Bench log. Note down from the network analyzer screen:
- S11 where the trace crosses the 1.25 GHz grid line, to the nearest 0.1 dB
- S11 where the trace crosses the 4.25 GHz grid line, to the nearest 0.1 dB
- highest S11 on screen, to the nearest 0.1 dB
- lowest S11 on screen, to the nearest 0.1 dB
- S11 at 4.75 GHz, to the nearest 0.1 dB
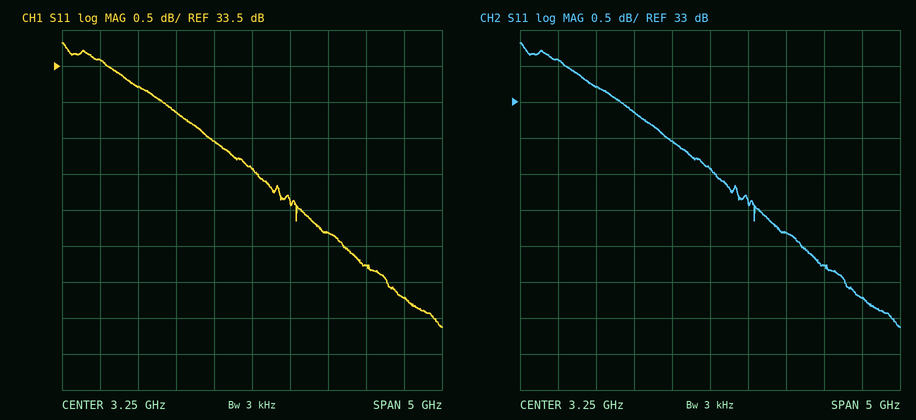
33.6 dB
31.2 dB
33.8 dB
29.9 dB
30.7 dB
